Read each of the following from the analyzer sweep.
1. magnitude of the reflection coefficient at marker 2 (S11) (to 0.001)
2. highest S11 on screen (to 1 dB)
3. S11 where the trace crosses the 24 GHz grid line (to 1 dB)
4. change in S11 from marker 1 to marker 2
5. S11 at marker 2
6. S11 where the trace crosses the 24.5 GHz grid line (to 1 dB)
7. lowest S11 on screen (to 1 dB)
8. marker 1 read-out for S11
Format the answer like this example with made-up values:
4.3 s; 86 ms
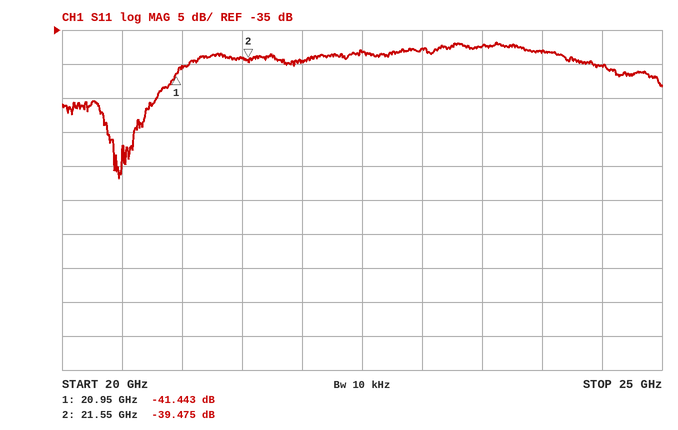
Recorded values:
0.011; -37 dB; -38 dB; 1.968 dB; -39.475 dB; -40 dB; -57 dB; -41.443 dB
